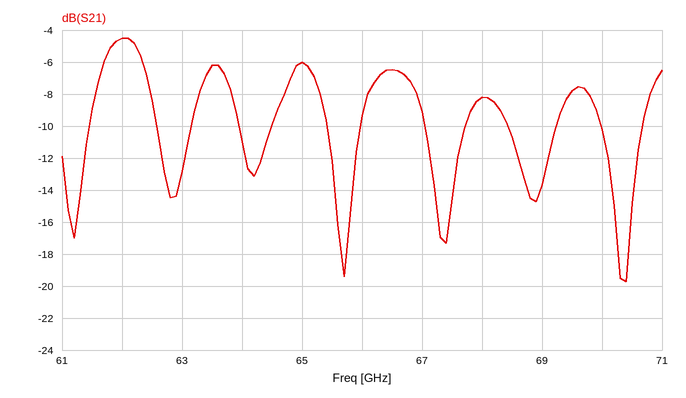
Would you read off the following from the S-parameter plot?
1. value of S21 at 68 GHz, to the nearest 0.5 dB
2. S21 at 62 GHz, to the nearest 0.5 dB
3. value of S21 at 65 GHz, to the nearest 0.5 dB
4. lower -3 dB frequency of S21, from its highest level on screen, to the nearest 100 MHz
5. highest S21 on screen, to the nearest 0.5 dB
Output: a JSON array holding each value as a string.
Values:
["-8.0 dB", "-4.5 dB", "-6.0 dB", "61.6 GHz", "-4.5 dB"]
